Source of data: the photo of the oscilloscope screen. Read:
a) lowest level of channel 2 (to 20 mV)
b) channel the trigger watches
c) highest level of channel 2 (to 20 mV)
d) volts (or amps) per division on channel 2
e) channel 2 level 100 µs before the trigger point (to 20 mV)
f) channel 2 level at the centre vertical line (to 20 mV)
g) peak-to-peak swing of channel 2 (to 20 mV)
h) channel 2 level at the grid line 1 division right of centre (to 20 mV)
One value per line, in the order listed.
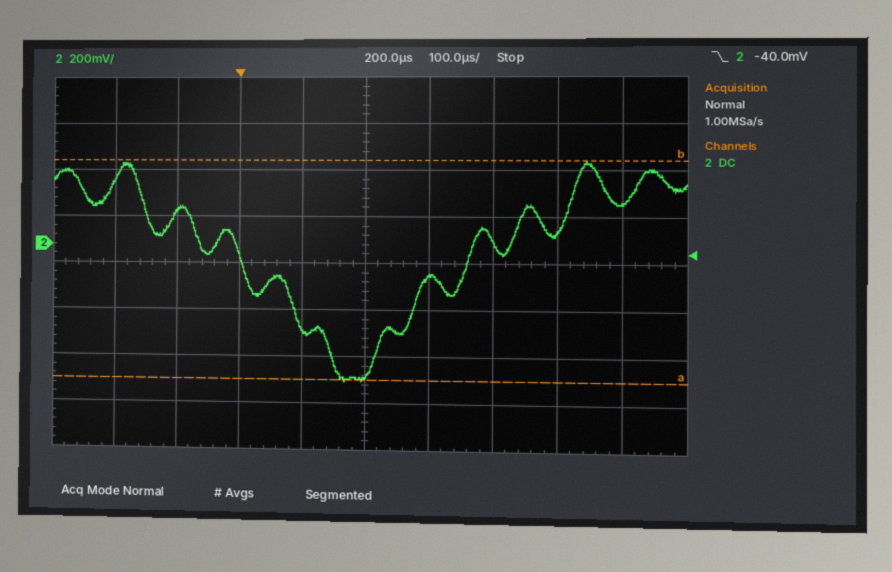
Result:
-580 mV
channel 2
360 mV
200 mV
140 mV
-560 mV
940 mV
-140 mV
